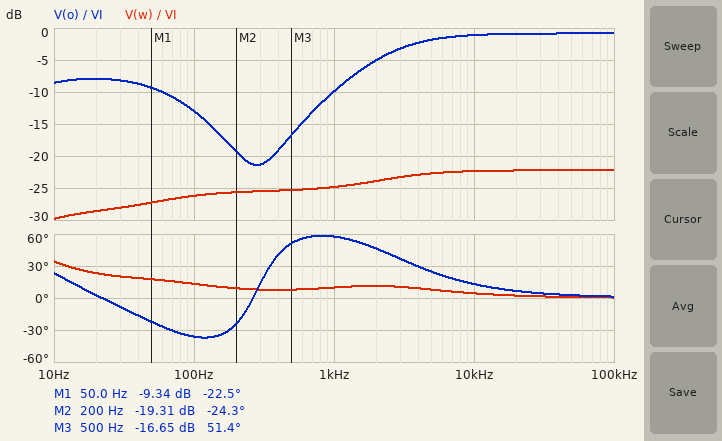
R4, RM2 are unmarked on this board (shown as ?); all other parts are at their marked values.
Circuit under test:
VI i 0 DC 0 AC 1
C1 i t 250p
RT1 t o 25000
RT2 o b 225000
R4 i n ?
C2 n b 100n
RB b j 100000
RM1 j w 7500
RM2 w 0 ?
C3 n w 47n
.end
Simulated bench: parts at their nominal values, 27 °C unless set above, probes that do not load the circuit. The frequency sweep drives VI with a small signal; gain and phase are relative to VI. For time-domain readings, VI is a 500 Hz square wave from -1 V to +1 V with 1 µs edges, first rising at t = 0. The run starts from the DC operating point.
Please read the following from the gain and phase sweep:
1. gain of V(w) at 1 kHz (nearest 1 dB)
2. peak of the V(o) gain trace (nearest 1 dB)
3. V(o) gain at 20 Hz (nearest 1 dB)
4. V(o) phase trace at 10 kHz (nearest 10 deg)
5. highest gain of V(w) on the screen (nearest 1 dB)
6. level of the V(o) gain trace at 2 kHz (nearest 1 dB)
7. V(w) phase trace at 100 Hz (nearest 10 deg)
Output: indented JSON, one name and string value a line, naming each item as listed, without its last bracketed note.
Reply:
{
  "gain of V(w) at 1 kHz": "-25 dB",
  "peak of the V(o) gain trace": "-1 dB",
  "V(o) gain at 20 Hz": "-8 dB",
  "V(o) phase trace at 10 kHz": "10 deg",
  "highest gain of V(w) on the screen": "-22 dB",
  "level of the V(o) gain trace at 2 kHz": "-5 dB",
  "V(w) phase trace at 100 Hz": "10 deg"
}
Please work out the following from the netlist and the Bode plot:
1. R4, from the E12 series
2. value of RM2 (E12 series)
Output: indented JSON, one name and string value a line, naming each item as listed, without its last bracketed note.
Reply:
{
  "R4, from the E12 series": "120 kΩ",
  "value of RM2": "6.8 kΩ"
}
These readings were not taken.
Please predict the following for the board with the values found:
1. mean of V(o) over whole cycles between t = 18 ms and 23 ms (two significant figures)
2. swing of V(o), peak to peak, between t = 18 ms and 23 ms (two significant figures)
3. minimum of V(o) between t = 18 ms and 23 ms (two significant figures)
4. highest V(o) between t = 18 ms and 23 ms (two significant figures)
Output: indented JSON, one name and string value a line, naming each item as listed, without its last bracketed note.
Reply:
{
  "mean of V(o) over whole cycles between t = 18 ms and 23 ms": "220 mV",
  "swing of V(o), peak to peak, between t = 18 ms and 23 ms": "3.4 V",
  "minimum of V(o) between t = 18 ms and 23 ms": "-1.5 V",
  "highest V(o) between t = 18 ms and 23 ms": "1.9 V"
}
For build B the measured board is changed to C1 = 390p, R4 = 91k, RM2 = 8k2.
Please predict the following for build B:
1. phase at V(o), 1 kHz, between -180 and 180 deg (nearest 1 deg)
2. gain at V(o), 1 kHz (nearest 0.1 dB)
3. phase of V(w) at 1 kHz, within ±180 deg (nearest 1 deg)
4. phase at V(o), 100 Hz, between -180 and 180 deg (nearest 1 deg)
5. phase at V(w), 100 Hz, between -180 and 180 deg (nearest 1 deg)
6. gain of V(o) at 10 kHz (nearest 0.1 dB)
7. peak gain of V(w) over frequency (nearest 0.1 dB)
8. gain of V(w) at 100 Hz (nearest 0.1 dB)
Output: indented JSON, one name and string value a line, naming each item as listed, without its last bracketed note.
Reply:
{
  "phase at V(o), 1 kHz, between -180 and 180 deg": "48 deg",
  "gain at V(o), 1 kHz": "-6.7 dB",
  "phase of V(w) at 1 kHz, within ±180 deg": "10 deg",
  "phase at V(o), 100 Hz, between -180 and 180 deg": "-30 deg",
  "phase at V(w), 100 Hz, between -180 and 180 deg": "16 deg",
  "gain of V(o) at 10 kHz": "-0.9 dB",
  "peak gain of V(w) over frequency": "-19.2 dB",
  "gain of V(w) at 100 Hz": "-22.7 dB"
}
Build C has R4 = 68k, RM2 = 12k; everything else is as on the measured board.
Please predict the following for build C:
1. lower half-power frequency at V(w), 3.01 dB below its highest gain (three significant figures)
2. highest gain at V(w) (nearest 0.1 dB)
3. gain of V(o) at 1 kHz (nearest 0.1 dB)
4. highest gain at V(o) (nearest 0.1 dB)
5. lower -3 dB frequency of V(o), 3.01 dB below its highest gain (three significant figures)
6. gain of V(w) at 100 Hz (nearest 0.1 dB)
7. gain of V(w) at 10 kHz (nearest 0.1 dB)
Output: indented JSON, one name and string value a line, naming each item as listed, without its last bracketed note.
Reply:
{
  "lower half-power frequency at V(w), 3.01 dB below its highest gain": "106 Hz",
  "highest gain at V(w)": "-14.7 dB",
  "gain of V(o) at 1 kHz": "-9.2 dB",
  "highest gain at V(o)": "-0.7 dB",
  "lower -3 dB frequency of V(o), 3.01 dB below its highest gain": "2.47 kHz",
  "gain of V(w) at 100 Hz": "-17.9 dB",
  "gain of V(w) at 10 kHz": "-14.8 dB"
}
